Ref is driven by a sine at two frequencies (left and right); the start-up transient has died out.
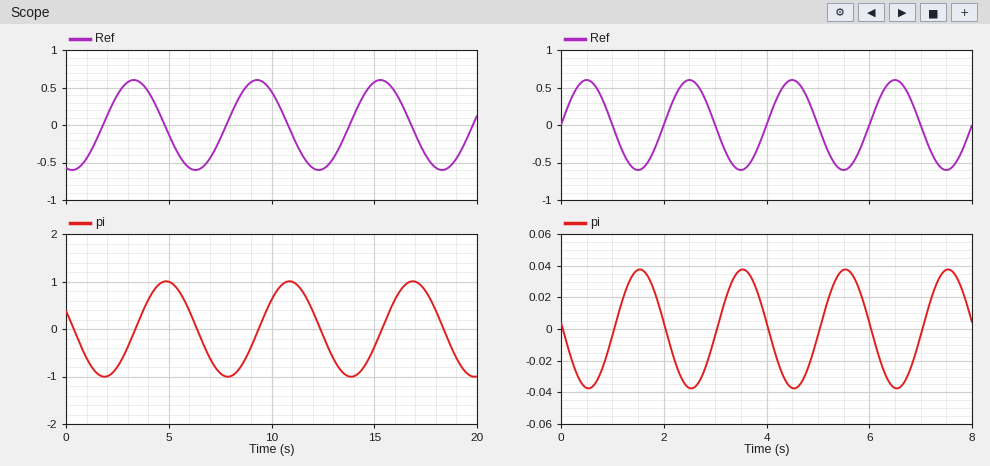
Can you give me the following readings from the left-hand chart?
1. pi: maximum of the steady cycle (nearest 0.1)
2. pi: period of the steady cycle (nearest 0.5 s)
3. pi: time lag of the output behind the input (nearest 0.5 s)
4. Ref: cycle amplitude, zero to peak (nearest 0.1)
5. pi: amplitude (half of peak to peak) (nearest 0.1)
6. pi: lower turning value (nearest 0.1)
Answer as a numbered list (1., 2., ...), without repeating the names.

1. 1.0
2. 6.0 s
3. 1.5 s
4. 0.6
5. 1.0
6. -1.0
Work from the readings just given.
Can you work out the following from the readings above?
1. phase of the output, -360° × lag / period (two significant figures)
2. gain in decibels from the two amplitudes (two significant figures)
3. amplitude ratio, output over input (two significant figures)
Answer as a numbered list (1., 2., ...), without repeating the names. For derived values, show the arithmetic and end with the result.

1. -360 × 1.5 / 6 = -90°
2. 20 log10(1 / 0.6) = 4.4 dB
3. 1 / 0.6 = 1.7
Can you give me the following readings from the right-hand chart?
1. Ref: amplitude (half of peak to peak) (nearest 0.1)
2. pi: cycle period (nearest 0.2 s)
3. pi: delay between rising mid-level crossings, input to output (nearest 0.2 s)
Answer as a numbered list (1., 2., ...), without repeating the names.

1. 0.6
2. 2.0 s
3. 1.0 s
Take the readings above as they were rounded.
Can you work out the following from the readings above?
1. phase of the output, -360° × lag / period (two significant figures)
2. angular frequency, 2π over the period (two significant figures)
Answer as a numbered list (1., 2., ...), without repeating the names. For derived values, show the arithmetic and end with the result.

1. -360 × 1 / 2 = -180°
2. 2π / 2 = 3.1 rad/s
